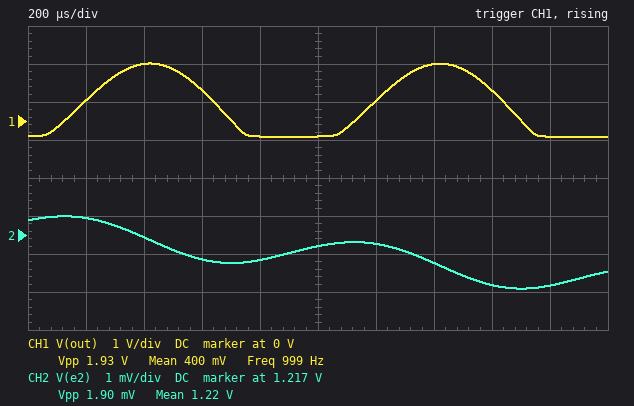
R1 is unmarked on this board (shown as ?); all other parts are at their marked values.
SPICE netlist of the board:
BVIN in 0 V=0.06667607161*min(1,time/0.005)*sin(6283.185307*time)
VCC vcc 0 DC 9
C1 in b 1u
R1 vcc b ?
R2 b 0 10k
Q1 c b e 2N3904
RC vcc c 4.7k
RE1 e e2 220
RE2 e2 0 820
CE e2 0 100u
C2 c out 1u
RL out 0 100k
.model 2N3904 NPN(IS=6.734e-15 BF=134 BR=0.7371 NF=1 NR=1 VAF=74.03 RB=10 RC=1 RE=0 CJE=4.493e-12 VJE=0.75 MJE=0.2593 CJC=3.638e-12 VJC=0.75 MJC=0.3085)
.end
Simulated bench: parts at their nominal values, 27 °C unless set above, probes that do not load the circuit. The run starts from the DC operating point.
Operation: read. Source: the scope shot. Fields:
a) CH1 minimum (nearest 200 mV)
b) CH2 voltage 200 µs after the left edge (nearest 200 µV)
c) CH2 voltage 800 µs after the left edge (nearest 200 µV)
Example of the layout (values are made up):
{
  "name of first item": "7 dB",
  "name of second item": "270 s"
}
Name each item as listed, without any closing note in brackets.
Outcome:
{
  "CH1 minimum": "-400 mV",
  "CH2 voltage 200 µs after the left edge": "1.2174 V",
  "CH2 voltage 800 µs after the left edge": "1.2164 V"
}
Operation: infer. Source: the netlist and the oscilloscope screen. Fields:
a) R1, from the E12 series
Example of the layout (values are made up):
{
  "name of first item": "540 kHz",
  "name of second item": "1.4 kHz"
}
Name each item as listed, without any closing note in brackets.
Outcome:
{
  "R1, from the E12 series": "27 kΩ"
}
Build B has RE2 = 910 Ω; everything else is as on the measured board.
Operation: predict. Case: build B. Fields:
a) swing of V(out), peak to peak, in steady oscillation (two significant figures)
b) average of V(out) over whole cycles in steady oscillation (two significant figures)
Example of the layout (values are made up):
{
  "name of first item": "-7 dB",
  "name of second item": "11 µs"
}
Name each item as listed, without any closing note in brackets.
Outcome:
{
  "swing of V(out), peak to peak, in steady oscillation": "2.1 V",
  "average of V(out) over whole cycles in steady oscillation": "330 mV"
}
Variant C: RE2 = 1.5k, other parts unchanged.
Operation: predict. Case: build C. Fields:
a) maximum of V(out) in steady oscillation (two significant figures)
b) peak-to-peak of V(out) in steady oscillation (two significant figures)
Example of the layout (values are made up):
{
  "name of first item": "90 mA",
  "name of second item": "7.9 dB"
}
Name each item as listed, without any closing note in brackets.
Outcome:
{
  "maximum of V(out) in steady oscillation": "1.2 V",
  "peak-to-peak of V(out) in steady oscillation": "2.4 V"
}
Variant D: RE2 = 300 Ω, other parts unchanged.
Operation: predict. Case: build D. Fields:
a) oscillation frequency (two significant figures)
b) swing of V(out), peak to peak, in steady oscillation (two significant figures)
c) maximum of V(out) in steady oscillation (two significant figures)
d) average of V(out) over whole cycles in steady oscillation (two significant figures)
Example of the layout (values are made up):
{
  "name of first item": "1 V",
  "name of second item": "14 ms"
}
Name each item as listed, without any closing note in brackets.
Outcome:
{
  "oscillation frequency": "1.0 kHz",
  "swing of V(out), peak to peak, in steady oscillation": "940 mV",
  "maximum of V(out) in steady oscillation": "810 mV",
  "average of V(out) over whole cycles in steady oscillation": "150 mV"
}
